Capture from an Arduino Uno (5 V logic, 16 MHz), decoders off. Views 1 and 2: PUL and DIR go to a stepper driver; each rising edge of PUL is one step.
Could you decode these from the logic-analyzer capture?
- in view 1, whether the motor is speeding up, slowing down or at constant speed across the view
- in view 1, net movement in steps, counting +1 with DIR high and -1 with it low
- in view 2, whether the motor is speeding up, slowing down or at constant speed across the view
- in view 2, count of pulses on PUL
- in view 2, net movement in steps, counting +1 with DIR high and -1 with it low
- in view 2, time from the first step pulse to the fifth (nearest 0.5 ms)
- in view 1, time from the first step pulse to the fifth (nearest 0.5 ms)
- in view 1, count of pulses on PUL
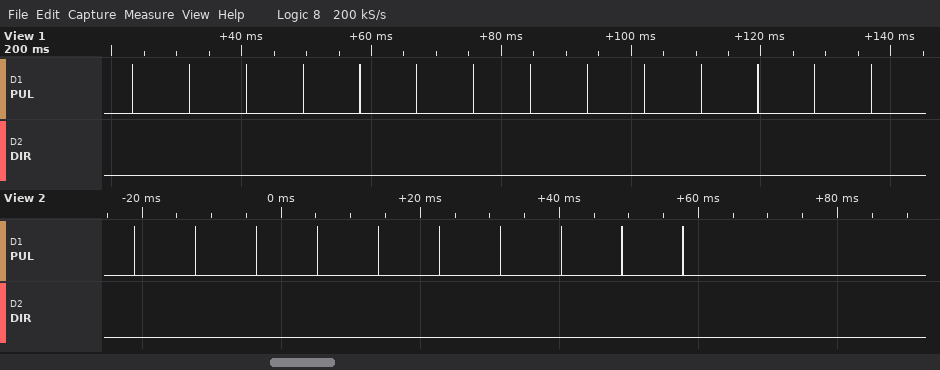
constant speed
-14
constant speed
10
-10
35.0 ms
35.0 ms
14
